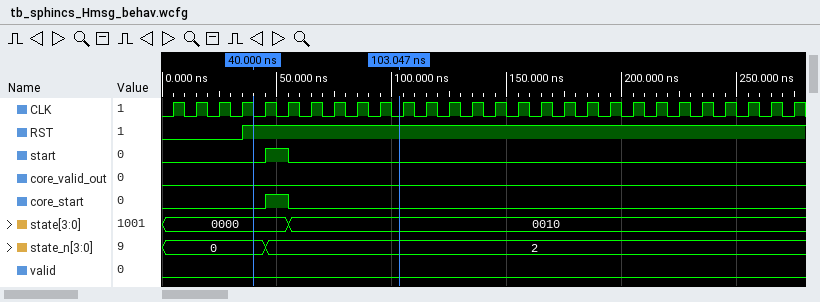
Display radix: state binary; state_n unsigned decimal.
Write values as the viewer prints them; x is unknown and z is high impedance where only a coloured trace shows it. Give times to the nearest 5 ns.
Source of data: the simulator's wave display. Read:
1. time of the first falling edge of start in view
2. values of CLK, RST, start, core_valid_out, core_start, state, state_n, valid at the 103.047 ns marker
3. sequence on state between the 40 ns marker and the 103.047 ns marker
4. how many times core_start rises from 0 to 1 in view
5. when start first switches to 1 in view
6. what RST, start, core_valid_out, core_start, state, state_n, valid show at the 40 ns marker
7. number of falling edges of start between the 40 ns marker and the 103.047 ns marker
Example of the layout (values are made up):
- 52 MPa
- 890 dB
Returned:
- 55 ns
- CLK=0, RST=1, start=0, core_valid_out=0, core_start=0, state=0010, state_n=2, valid=0
- 0000, 0010
- 1
- 45 ns
- RST=1, start=0, core_valid_out=0, core_start=0, state=0000, state_n=0, valid=0
- 1
